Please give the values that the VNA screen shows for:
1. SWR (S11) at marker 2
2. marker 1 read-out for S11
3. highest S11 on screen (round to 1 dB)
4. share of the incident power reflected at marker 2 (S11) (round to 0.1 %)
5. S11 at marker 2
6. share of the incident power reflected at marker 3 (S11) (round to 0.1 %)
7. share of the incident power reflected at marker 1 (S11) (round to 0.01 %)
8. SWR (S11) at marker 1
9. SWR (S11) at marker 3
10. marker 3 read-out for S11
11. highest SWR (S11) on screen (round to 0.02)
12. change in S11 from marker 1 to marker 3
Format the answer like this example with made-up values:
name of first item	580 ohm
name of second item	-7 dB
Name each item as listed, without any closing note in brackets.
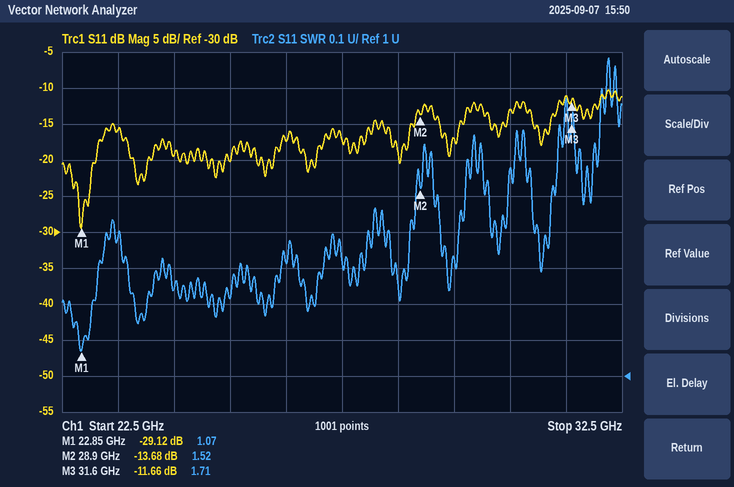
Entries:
SWR (S11) at marker 2	1.52
marker 1 read-out for S11	-29.12 dB
highest S11 on screen	-10 dB
share of the incident power reflected at marker 2 (S11)	4.3 %
S11 at marker 2	-13.68 dB
share of the incident power reflected at marker 3 (S11)	6.8 %
share of the incident power reflected at marker 1 (S11)	0.12 %
SWR (S11) at marker 1	1.07
SWR (S11) at marker 3	1.71
marker 3 read-out for S11	-11.66 dB
highest SWR (S11) on screen	1.88
change in S11 from marker 1 to marker 3	17.46 dB
